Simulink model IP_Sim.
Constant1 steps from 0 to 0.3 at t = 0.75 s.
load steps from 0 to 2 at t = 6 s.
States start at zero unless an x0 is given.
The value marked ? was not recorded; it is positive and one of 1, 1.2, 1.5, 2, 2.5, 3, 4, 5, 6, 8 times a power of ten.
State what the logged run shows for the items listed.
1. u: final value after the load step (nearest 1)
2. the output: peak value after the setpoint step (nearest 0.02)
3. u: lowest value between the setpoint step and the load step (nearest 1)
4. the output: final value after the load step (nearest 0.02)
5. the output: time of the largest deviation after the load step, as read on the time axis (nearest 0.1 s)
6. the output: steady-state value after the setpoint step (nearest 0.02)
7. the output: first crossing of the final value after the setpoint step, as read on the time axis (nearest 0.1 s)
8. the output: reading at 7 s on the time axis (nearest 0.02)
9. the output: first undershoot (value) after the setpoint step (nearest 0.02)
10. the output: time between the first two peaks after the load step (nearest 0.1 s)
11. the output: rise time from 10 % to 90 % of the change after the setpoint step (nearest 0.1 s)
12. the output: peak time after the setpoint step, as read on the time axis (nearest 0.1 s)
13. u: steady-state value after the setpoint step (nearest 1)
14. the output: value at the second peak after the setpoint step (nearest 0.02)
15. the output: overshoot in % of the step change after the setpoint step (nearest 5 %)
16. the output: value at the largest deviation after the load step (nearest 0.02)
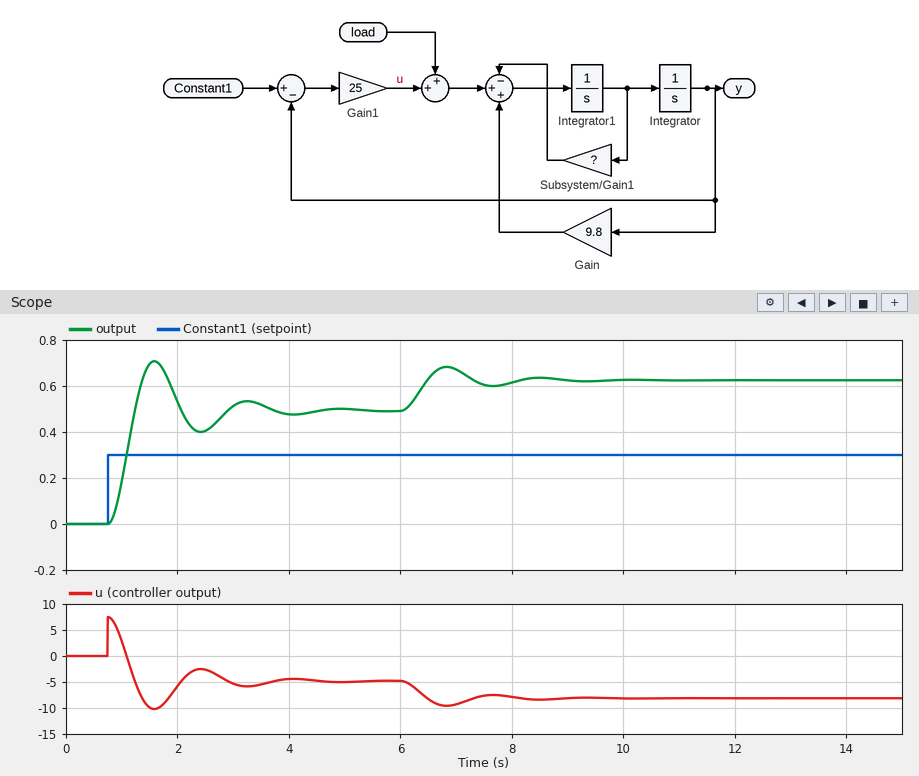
-8
0.70
-10
0.62
6.8 s
0.50
1.2 s
0.68
0.40
1.7 s
0.3 s
1.6 s
-5
0.54
45 %
0.68
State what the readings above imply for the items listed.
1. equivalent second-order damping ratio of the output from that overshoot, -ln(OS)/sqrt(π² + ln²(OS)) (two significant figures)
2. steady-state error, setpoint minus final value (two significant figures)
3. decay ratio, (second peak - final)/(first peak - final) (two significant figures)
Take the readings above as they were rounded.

0.25
-0.20
0.20
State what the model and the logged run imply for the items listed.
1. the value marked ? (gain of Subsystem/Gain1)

2
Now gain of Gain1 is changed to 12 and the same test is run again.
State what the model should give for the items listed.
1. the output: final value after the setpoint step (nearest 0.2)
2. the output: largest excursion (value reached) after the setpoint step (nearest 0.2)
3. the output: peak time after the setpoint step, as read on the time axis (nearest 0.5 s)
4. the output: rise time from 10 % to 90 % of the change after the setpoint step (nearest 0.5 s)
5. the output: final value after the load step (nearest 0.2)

1.6
1.8
3.5 s
1.5 s
2.6
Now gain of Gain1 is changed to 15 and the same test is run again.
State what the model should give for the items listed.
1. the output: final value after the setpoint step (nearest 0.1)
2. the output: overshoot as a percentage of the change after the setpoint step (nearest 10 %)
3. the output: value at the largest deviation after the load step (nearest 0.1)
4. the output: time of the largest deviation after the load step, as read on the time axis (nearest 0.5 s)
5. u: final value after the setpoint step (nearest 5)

0.9
20 %
1.3
7.5 s
-10
